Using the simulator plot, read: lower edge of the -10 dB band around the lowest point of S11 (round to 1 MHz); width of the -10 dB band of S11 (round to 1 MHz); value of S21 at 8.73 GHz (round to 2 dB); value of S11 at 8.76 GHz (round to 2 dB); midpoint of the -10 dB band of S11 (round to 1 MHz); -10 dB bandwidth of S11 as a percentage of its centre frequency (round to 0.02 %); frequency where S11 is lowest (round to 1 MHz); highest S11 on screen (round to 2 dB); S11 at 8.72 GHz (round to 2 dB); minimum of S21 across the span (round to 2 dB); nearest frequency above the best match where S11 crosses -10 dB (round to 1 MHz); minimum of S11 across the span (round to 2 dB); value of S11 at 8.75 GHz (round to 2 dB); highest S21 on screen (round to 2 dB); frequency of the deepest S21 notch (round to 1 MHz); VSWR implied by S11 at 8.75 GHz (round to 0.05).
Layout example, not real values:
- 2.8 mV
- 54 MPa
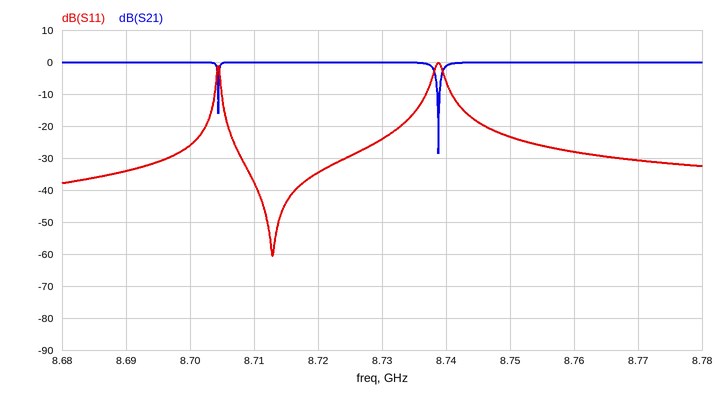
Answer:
- 8.705 GHz
- 32 MHz
- 0 dB
- -28 dB
- 8.721 GHz
- 0.36 %
- 8.713 GHz
- 0 dB
- -34 dB
- -28 dB
- 8.737 GHz
- -60 dB
- -24 dB
- 0 dB
- 8.739 GHz
- 1.15
